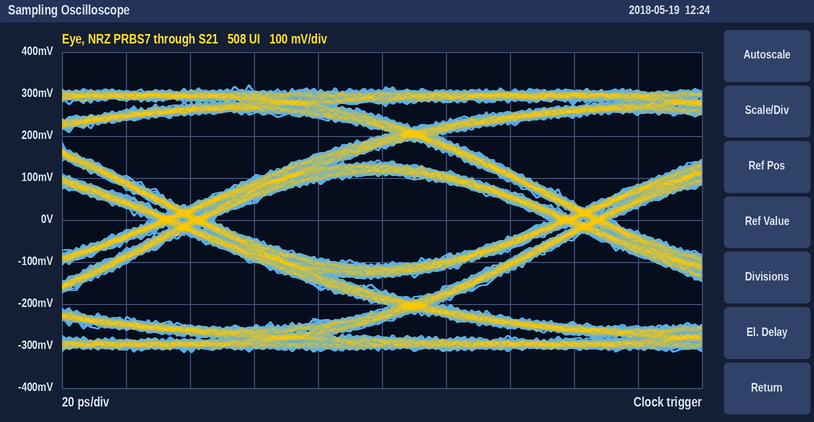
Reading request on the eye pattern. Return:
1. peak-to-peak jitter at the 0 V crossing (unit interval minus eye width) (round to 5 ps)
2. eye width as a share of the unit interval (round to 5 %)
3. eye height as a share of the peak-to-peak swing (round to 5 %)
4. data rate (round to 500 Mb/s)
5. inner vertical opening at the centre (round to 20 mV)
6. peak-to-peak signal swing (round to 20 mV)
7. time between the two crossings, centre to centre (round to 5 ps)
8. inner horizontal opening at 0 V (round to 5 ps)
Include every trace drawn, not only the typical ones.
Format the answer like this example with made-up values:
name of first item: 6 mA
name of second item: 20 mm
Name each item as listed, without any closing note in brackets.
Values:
peak-to-peak jitter at the 0 V crossing (unit interval minus eye width): 20 ps
eye width as a share of the unit interval: 85 %
eye height as a share of the peak-to-peak swing: 35 %
data rate: 8.0 Gb/s
inner vertical opening at the centre: 220 mV
peak-to-peak signal swing: 640 mV
time between the two crossings, centre to centre: 125 ps
inner horizontal opening at 0 V: 105 ps
